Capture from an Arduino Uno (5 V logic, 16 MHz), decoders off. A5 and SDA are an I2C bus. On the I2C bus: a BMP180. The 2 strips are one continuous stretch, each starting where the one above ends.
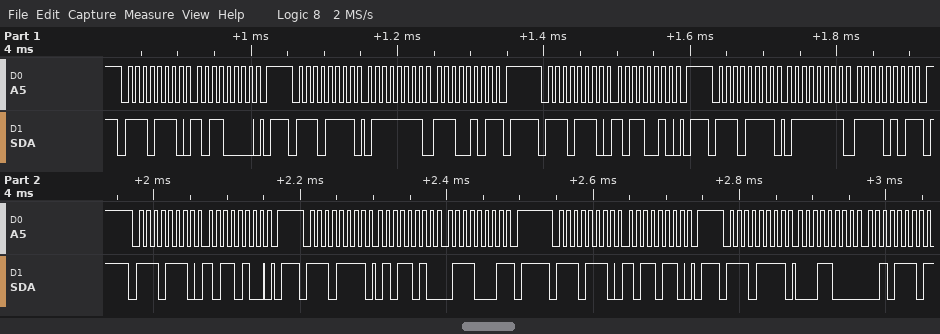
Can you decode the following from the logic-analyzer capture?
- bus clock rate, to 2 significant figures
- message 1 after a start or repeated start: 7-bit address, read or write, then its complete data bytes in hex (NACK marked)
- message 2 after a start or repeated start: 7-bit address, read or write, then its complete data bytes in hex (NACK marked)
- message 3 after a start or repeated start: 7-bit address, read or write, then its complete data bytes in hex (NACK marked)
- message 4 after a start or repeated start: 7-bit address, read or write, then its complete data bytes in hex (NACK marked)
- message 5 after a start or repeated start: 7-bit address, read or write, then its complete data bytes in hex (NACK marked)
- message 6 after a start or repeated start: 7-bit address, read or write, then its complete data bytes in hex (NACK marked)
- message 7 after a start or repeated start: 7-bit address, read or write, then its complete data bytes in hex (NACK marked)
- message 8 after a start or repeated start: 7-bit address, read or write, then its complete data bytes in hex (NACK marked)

100 kHz
0x77 write: B0
0x77 read: 7F E5 NACK
0x77 write: B2
0x77 read: 7F F5 NACK
0x77 write: B4
0x77 read: 5A 71 NACK
0x77 write: B6
0x77 read: 18 2E NACK
